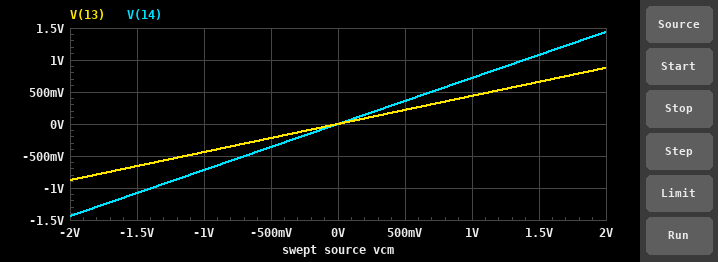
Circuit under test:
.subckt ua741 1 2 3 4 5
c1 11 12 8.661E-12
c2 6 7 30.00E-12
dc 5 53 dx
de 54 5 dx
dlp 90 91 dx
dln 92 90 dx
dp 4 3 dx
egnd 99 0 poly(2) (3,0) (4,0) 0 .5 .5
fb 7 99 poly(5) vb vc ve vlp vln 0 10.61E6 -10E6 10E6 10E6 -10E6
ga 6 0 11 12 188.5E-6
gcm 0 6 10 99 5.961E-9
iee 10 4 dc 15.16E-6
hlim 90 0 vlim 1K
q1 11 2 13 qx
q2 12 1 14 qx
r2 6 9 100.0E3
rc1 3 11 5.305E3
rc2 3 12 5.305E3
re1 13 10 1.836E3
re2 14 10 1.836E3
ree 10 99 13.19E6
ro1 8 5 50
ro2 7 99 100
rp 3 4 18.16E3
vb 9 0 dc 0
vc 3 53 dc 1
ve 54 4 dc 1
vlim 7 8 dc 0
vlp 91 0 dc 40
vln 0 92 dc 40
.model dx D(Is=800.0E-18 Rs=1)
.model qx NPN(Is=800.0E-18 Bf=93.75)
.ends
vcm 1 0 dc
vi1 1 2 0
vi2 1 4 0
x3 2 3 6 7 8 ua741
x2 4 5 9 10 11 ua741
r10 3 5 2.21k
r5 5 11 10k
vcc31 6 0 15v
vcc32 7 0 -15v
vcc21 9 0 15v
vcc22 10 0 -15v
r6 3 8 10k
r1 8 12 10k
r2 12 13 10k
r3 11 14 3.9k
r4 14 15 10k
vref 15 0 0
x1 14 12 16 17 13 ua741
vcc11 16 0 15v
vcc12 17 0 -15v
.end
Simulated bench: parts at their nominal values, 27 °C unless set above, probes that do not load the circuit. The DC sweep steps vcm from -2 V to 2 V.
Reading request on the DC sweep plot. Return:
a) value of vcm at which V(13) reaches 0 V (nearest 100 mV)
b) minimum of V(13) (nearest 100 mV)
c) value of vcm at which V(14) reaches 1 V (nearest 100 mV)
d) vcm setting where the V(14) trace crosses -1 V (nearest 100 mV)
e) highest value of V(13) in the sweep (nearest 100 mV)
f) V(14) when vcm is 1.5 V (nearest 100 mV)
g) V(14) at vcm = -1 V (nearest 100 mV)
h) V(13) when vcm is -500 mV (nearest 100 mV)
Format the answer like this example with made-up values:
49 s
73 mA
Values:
0 V
-900 mV
1.4 V
-1.4 V
900 mV
1.1 V
-700 mV
-200 mV
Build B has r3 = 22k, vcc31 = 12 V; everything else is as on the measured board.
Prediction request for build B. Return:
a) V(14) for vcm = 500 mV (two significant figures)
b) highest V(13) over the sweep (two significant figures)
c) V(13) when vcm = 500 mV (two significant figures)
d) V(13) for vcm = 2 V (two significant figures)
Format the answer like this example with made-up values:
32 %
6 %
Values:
160 mV
750 mV
-190 mV
-750 mV
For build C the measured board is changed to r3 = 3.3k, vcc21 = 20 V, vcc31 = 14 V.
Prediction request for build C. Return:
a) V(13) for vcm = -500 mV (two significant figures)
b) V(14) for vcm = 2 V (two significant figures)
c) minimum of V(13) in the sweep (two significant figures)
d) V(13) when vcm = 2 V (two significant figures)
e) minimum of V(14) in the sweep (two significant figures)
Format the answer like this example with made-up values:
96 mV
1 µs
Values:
-250 mV
1.5 V
-1.0 V
1.0 V
-1.5 V
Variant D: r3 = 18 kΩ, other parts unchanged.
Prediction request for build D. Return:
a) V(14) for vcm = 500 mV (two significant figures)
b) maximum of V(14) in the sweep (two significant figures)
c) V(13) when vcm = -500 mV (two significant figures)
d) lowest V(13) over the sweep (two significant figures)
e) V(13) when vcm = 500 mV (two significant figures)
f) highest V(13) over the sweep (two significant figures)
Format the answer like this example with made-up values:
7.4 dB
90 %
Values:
180 mV
710 mV
140 mV
-570 mV
-140 mV
570 mV
